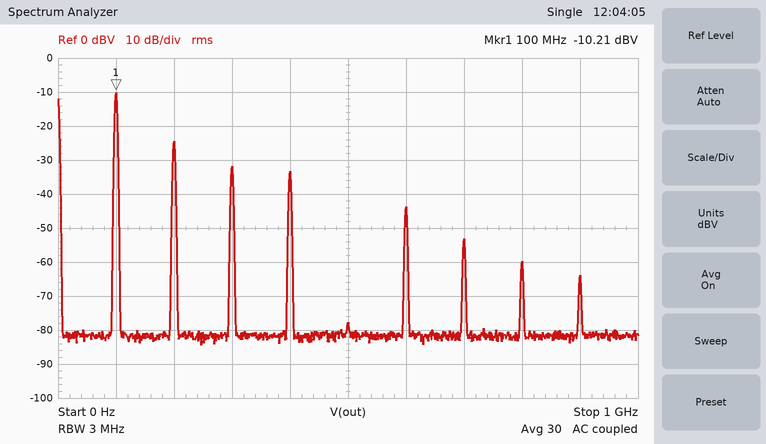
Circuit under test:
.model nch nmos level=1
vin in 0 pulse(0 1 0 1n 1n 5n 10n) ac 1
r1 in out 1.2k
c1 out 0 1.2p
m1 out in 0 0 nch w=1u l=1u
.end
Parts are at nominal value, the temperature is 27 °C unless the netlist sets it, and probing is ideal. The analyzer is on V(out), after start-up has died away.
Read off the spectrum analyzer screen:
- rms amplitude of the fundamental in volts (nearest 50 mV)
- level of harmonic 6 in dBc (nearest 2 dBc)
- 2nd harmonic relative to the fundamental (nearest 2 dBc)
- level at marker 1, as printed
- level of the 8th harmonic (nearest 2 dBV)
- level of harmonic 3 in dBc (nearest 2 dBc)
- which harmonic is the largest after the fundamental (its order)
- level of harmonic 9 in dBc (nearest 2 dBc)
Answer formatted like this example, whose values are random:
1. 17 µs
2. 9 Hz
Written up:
1. 300 mV
2. -34 dBc
3. -14 dBc
4. -10.21 dBV
5. -60 dBV
6. -22 dBc
7. 2
8. -54 dBc
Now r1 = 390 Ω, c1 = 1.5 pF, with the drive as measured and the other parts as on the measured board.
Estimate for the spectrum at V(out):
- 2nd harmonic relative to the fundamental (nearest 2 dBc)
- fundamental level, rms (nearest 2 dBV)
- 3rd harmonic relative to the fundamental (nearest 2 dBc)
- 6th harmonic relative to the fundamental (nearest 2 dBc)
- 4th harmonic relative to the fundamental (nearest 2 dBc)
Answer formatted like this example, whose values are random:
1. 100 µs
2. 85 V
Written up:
1. -12 dBc
2. -8 dBV
3. -18 dBc
4. -28 dBc
5. -18 dBc
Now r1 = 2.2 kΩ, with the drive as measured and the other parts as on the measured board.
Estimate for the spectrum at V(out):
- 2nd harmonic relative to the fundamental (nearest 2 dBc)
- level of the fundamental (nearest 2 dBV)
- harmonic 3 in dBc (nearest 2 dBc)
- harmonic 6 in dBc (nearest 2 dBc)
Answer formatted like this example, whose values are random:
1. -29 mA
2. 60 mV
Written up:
1. -16 dBc
2. -14 dBV
3. -24 dBc
4. -36 dBc
